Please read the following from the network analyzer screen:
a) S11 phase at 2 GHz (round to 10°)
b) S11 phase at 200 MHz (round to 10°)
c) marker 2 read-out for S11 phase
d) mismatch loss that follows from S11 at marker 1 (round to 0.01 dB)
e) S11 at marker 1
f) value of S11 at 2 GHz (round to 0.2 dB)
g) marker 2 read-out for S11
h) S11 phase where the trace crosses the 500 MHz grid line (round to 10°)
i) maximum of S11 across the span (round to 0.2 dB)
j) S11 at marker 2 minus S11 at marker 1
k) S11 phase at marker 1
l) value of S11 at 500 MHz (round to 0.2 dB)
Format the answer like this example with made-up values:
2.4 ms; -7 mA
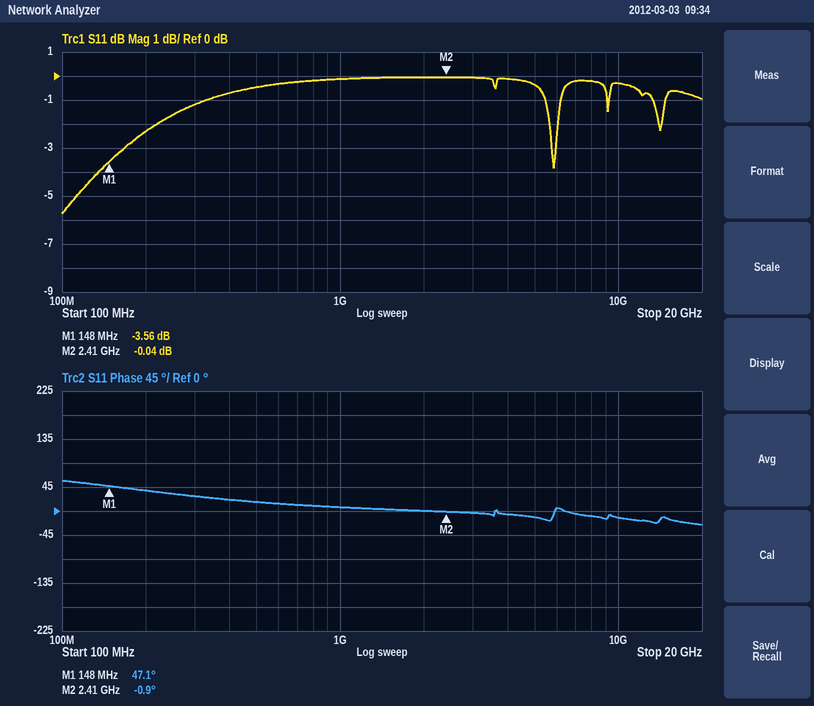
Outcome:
0°; 40°; -0.9°; 2.52 dB; -3.56 dB; 0.0 dB; -0.04 dB; 20°; 0.0 dB; 3.52 dB; 47.1°; -0.4 dB
